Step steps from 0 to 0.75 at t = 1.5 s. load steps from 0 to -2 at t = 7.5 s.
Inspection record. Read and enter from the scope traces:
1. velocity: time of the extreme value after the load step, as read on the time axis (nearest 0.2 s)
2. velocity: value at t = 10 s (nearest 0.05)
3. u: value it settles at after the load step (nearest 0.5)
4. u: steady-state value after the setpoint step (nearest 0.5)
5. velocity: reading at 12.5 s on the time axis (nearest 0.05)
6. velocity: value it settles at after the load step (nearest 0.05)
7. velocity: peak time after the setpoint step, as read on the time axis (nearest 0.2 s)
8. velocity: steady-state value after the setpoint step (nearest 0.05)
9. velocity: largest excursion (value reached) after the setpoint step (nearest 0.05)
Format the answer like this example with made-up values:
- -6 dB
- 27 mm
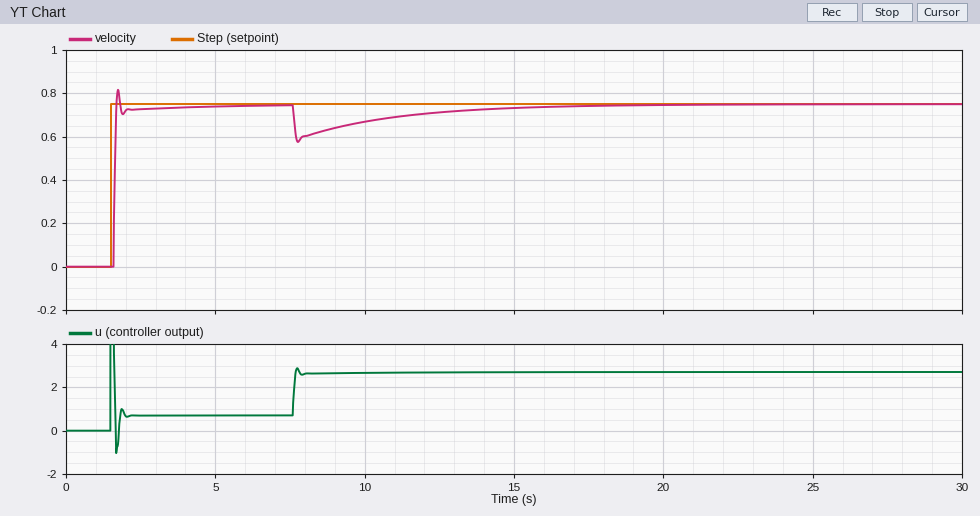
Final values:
- 7.8 s
- 0.65
- 2.5
- 0.5
- 0.70
- 0.75
- 1.8 s
- 0.75
- 0.80
